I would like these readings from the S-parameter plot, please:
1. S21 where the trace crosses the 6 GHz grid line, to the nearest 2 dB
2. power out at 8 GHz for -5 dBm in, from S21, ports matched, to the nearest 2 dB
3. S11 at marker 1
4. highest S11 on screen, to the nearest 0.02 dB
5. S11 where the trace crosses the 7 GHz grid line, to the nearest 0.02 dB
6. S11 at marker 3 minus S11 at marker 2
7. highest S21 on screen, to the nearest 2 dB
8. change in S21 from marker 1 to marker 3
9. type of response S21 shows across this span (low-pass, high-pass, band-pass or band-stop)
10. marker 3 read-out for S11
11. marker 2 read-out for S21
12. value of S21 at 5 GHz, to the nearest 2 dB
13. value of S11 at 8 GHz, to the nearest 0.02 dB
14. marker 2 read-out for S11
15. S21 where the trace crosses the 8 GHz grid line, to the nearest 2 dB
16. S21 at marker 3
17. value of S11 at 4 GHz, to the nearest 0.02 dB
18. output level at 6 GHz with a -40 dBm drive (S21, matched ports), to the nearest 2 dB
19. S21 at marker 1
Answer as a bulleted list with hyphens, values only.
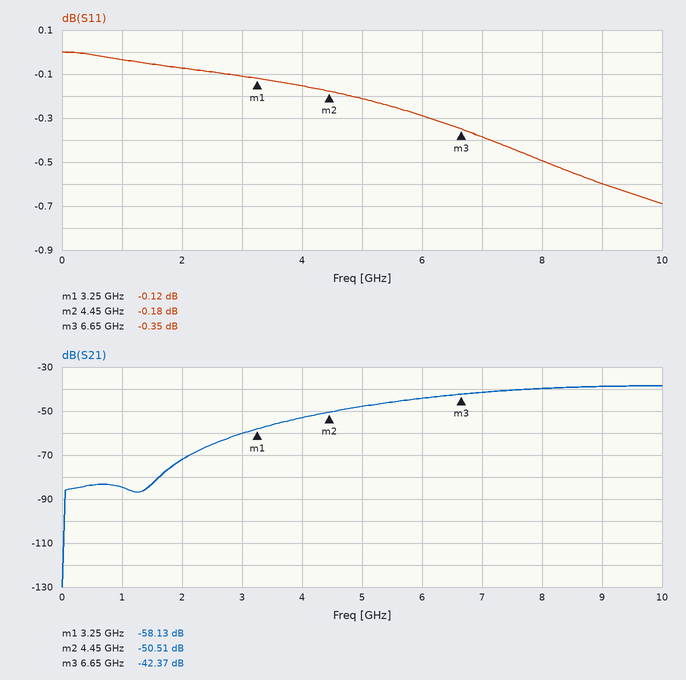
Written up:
- -44 dB
- -44 dBm
- -0.12 dB
- 0.00 dB
- -0.38 dB
- -0.17 dB
- -38 dB
- 15.76 dB
- high-pass
- -0.35 dB
- -50.51 dB
- -48 dB
- -0.50 dB
- -0.18 dB
- -40 dB
- -42.37 dB
- -0.16 dB
- -84 dBm
- -58.13 dB
